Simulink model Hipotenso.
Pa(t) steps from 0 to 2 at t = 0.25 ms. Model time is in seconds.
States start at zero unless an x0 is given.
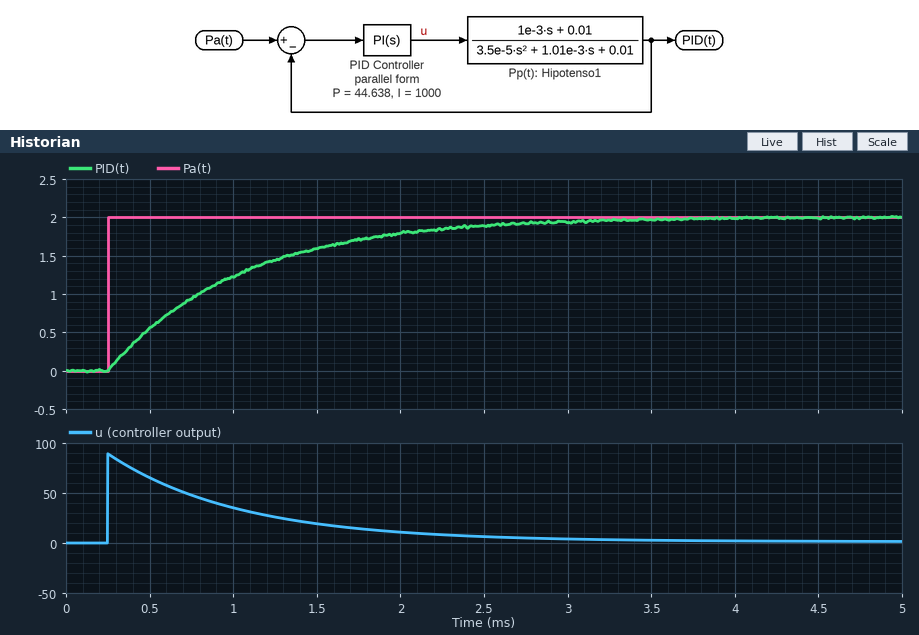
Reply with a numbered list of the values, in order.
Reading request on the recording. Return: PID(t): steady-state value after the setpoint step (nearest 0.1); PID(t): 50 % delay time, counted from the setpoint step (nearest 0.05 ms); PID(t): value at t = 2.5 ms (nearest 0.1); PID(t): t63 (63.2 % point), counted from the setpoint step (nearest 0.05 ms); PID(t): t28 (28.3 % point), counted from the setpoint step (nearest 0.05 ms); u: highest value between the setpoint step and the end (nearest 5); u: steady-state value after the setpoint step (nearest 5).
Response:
1. 2.0
2. 0.55 ms
3. 1.9
4. 0.80 ms
5. 0.25 ms
6. 90
7. 0
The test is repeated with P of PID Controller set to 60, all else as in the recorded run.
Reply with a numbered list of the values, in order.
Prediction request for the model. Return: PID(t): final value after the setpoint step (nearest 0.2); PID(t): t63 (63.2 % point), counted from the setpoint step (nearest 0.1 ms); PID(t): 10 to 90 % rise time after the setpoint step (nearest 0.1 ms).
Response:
1. 2.0
2. 0.6 ms
3. 1.3 ms
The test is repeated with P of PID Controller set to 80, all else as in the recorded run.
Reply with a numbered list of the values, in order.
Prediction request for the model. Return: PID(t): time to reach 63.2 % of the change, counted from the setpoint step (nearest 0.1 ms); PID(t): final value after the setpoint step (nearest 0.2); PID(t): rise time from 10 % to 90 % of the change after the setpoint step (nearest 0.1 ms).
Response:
1. 0.4 ms
2. 2.0
3. 1.0 ms
